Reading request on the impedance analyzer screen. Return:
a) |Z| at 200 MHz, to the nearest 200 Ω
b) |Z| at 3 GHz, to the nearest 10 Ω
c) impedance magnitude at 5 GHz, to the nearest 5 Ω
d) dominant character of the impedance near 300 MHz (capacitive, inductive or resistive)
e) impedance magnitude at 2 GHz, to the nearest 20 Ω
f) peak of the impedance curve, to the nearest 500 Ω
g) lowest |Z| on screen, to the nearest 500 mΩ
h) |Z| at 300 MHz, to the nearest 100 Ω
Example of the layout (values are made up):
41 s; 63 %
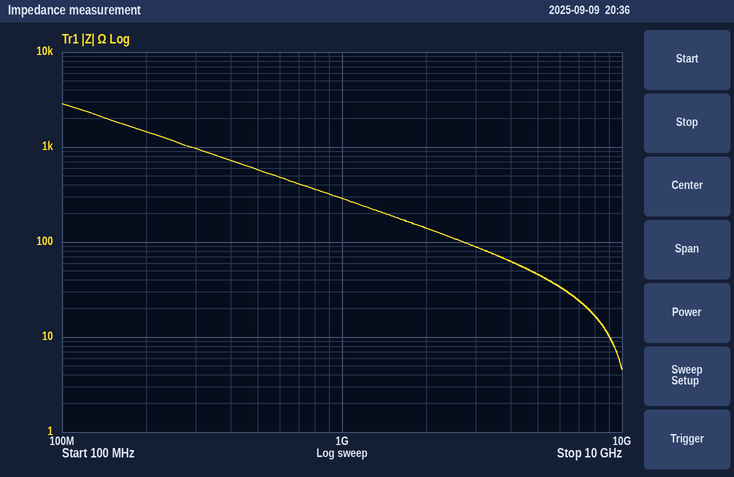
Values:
1.4 kΩ; 90 Ω; 45 Ω; capacitive; 140 Ω; 3.0 kΩ; 4.5 Ω; 1.0 kΩ
